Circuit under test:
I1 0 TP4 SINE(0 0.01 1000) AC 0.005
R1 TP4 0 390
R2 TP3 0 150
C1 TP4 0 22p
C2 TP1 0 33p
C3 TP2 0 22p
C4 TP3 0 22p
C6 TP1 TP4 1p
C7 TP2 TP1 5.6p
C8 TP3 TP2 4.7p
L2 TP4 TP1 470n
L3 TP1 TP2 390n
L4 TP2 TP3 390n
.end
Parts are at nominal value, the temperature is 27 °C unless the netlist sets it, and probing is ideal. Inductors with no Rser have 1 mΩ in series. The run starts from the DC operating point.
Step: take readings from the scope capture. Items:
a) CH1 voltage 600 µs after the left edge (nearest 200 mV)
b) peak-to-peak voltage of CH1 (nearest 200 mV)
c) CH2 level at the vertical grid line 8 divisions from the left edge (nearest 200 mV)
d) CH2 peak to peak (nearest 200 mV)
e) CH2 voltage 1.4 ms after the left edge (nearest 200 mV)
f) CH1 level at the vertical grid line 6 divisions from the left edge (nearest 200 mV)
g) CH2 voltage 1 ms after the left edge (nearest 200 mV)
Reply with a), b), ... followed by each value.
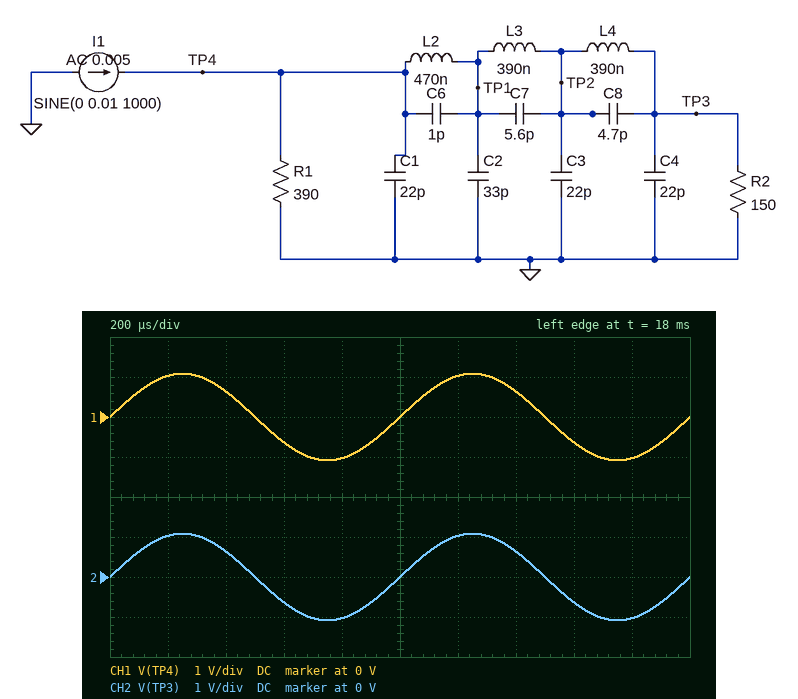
a) -600 mV
b) 2.2 V
c) -600 mV
d) 2.2 V
e) 600 mV
f) 1.0 V
g) 0 V
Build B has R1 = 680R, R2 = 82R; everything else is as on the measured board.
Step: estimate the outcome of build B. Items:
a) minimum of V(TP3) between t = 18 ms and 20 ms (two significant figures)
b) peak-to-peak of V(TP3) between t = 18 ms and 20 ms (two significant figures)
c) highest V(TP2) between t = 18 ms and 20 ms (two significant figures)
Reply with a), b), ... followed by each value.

a) -730 mV
b) 1.5 V
c) 730 mV
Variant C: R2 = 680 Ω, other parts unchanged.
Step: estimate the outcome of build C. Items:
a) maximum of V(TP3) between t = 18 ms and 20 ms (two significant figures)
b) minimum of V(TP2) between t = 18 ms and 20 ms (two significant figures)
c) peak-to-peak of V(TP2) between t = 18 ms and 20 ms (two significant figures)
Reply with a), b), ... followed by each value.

a) 2.5 V
b) -2.5 V
c) 5.0 V
